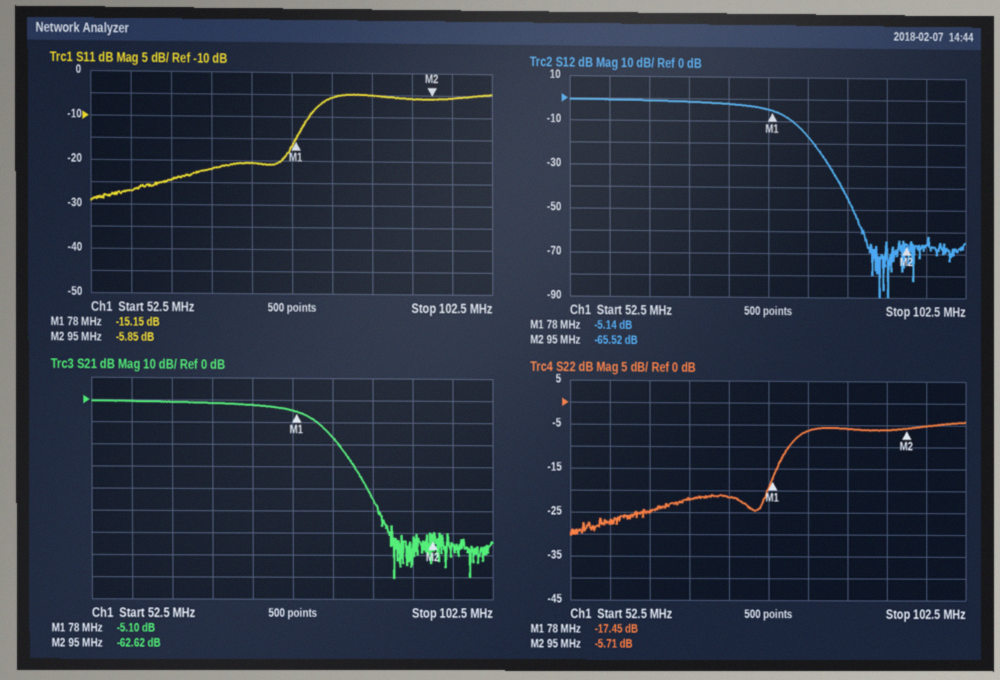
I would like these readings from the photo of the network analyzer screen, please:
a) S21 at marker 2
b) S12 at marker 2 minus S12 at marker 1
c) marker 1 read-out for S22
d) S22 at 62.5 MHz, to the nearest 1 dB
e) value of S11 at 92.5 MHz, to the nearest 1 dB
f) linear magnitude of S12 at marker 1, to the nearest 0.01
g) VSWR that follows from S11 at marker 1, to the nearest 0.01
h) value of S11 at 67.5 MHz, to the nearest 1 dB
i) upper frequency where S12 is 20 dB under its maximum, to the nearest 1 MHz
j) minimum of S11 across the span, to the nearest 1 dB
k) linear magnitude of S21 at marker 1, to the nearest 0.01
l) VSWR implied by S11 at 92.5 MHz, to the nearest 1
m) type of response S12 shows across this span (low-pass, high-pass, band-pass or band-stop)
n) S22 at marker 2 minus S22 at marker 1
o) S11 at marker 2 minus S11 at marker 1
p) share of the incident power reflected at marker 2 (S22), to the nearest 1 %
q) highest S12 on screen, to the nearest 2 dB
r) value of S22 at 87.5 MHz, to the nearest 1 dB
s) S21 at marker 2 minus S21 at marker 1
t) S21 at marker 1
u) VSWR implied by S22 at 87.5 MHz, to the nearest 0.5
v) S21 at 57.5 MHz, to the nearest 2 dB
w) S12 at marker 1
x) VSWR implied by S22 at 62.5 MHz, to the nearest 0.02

-62.62 dB
-60.38 dB
-17.45 dB
-25 dB
-6 dB
0.55
1.42
-22 dB
83 MHz
-29 dB
0.56
3
low-pass
11.74 dB
9.30 dB
27 %
0 dB
-6 dB
-57.52 dB
-5.10 dB
3.0
0 dB
-5.14 dB
1.12
